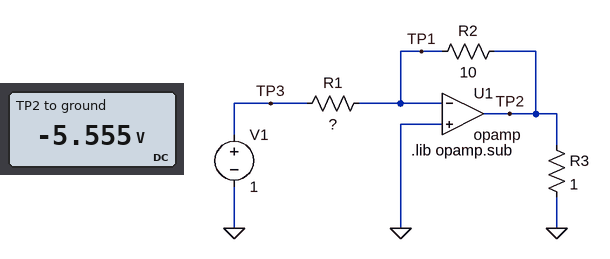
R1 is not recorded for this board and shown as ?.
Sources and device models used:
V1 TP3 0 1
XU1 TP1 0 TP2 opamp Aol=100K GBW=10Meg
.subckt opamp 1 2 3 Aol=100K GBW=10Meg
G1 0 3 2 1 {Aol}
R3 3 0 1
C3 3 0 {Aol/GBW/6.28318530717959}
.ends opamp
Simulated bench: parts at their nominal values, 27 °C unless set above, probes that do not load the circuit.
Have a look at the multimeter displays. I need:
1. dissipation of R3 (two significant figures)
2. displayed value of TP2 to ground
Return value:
31 W
-5.555 V
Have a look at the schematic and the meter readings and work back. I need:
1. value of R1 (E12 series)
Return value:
1.8 Ω
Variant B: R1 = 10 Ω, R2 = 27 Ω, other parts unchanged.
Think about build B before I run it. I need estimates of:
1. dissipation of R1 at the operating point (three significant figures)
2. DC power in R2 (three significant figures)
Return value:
100 mW
270 mW
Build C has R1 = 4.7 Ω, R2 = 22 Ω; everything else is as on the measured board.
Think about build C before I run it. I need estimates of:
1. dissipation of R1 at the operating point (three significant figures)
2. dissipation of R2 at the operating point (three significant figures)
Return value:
213 mW
996 mW
